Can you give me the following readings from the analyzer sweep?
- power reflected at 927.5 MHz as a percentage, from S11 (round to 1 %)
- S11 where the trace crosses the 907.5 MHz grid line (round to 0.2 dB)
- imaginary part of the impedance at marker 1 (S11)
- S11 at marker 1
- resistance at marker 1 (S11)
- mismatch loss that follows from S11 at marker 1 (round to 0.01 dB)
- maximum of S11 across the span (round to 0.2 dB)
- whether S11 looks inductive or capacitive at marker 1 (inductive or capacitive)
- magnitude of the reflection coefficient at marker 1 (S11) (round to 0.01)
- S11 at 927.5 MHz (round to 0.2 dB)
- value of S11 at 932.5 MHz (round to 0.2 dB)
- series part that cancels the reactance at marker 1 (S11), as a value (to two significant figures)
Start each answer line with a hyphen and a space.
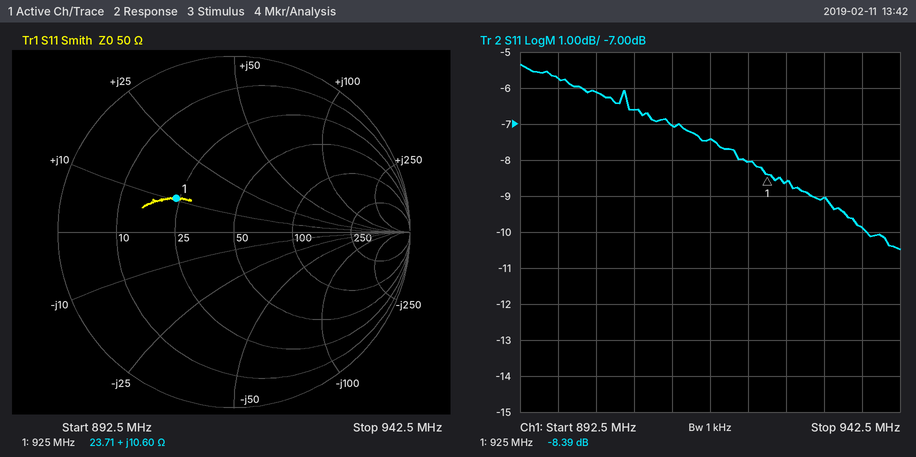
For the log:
- 14 %
- -6.6 dB
- +10.60 Ω
- -8.39 dB
- 23.71 Ω
- 0.68 dB
- -5.4 dB
- inductive
- 0.38
- -8.6 dB
- -9.0 dB
- 16 pF
